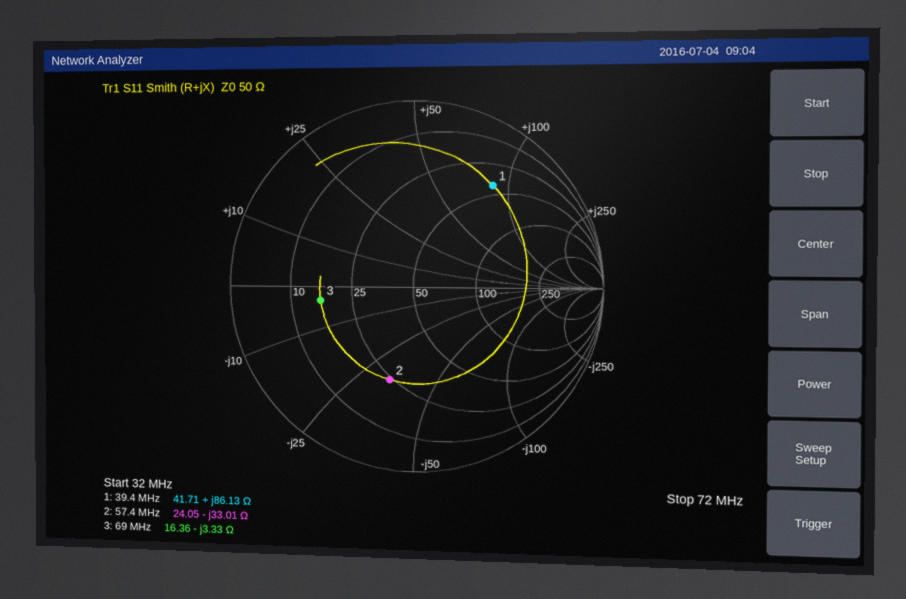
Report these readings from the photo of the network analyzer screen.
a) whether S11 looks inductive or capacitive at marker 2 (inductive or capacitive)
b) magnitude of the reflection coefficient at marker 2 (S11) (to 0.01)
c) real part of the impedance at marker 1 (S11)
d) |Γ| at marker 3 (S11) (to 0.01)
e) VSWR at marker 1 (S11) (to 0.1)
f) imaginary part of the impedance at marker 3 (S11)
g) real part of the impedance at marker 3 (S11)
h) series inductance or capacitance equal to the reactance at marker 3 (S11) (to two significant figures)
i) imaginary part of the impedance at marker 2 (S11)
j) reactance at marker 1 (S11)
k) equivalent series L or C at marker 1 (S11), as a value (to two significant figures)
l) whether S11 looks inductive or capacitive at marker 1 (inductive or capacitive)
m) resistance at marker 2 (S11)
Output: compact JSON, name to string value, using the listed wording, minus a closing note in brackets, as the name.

{"whether S11 looks inductive or capacitive at marker 2": "capacitive", "magnitude of the reflection coefficient at marker 2 (S11)": "0.52", "real part of the impedance at marker 1": "41.71 Ω", "|Γ| at marker 3 (S11)": "0.51", "VSWR at marker 1 (S11)": "5.4", "imaginary part of the impedance at marker 3": "-3.33 Ω", "real part of the impedance at marker 3": "16.36 Ω", "series inductance or capacitance equal to the reactance at marker 3 (S11)": "690 pF", "imaginary part of the impedance at marker 2": "-33.01 Ω", "reactance at marker 1": "+86.13 Ω", "equivalent series L or C at marker 1 (S11), as a value": "350 nH", "whether S11 looks inductive or capacitive at marker 1": "inductive", "resistance at marker 2": "24.05 Ω"}
